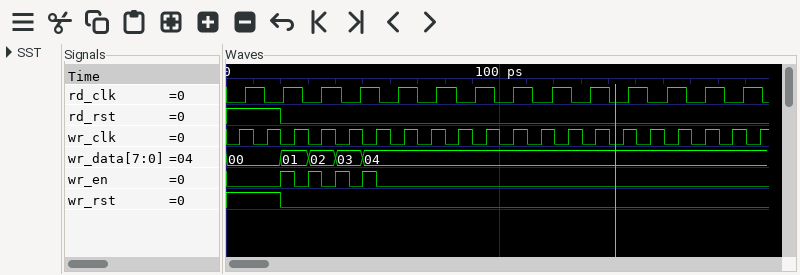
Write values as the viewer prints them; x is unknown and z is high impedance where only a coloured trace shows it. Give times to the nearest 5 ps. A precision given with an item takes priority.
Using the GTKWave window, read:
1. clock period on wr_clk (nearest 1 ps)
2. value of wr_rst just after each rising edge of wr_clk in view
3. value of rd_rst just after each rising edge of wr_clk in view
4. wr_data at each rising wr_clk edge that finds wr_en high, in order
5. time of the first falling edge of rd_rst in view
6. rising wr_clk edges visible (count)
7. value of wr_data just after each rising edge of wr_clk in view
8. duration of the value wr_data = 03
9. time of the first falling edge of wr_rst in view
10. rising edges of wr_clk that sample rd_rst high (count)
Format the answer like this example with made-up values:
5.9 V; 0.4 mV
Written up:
10 ps; 1 1 0 0 0 0 0 0 0 0 0 0 0 0 0 0 0 0 0 0; 1 1 0 0 0 0 0 0 0 0 0 0 0 0 0 0 0 0 0 0; 01, 02, 03, 04; 20 ps; 20; 00, 00, 01, 02, 03, 04, 04, 04, 04, 04, 04, 04, 04, 04, 04, 04, 04, 04, 04, 04; 10 ps; 20 ps; 2
